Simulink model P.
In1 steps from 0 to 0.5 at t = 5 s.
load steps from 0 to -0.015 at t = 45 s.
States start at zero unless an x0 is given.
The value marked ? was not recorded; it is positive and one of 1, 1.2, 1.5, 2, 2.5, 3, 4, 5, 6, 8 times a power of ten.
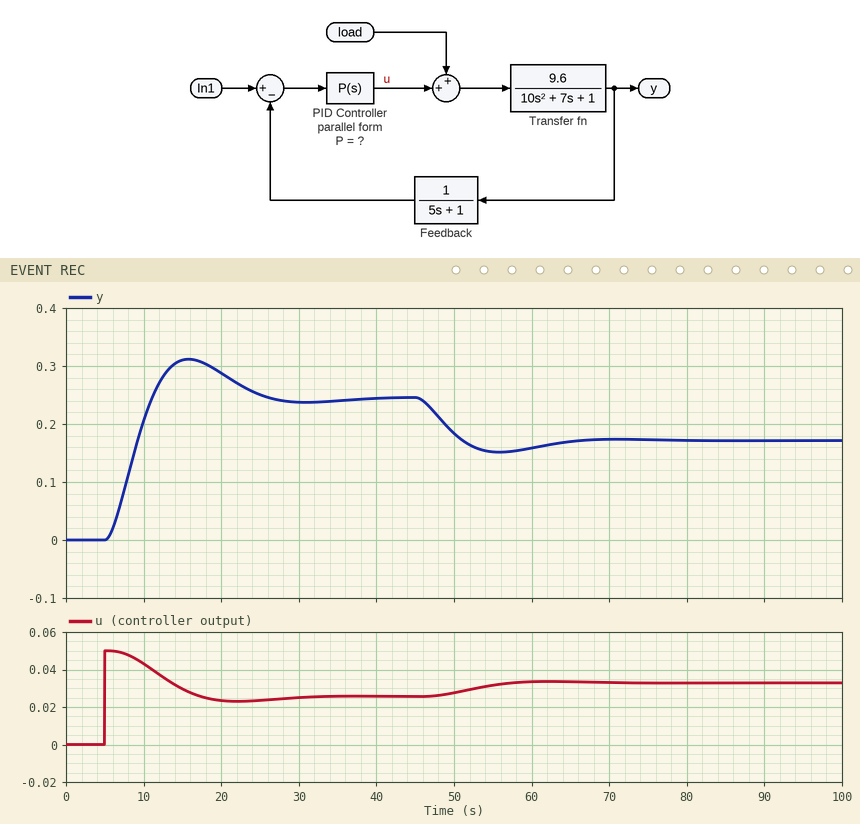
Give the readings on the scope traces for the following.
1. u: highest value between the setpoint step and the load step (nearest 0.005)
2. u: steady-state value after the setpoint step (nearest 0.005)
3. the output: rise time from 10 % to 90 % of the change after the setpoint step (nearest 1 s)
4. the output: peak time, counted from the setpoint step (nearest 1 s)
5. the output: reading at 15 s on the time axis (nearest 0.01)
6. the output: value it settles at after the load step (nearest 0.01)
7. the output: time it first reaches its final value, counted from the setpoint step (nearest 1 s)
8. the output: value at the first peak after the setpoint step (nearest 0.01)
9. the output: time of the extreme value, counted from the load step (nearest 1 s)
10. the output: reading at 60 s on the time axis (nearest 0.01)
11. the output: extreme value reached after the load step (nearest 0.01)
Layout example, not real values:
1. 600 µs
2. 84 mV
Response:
1. 0.050
2. 0.025
3. 4 s
4. 11 s
5. 0.31
6. 0.17
7. 6 s
8. 0.31
9. 11 s
10. 0.16
11. 0.15
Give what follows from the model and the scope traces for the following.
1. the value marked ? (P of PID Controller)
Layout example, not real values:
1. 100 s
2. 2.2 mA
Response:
1. 0.1
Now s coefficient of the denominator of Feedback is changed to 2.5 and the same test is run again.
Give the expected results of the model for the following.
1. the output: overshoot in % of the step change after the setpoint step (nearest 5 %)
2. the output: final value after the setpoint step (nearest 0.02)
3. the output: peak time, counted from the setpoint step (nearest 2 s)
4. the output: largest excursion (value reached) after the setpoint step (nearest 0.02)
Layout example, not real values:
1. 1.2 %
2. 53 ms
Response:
1. 15 %
2. 0.24
3. 10 s
4. 0.28
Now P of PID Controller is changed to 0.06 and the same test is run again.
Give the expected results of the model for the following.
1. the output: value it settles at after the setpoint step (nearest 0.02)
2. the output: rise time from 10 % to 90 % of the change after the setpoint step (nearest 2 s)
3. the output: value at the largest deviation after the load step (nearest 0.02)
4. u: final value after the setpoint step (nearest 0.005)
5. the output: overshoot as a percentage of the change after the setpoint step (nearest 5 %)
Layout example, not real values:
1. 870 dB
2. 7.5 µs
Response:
1. 0.18
2. 6 s
3. 0.08
4. 0.020
5. 15 %
